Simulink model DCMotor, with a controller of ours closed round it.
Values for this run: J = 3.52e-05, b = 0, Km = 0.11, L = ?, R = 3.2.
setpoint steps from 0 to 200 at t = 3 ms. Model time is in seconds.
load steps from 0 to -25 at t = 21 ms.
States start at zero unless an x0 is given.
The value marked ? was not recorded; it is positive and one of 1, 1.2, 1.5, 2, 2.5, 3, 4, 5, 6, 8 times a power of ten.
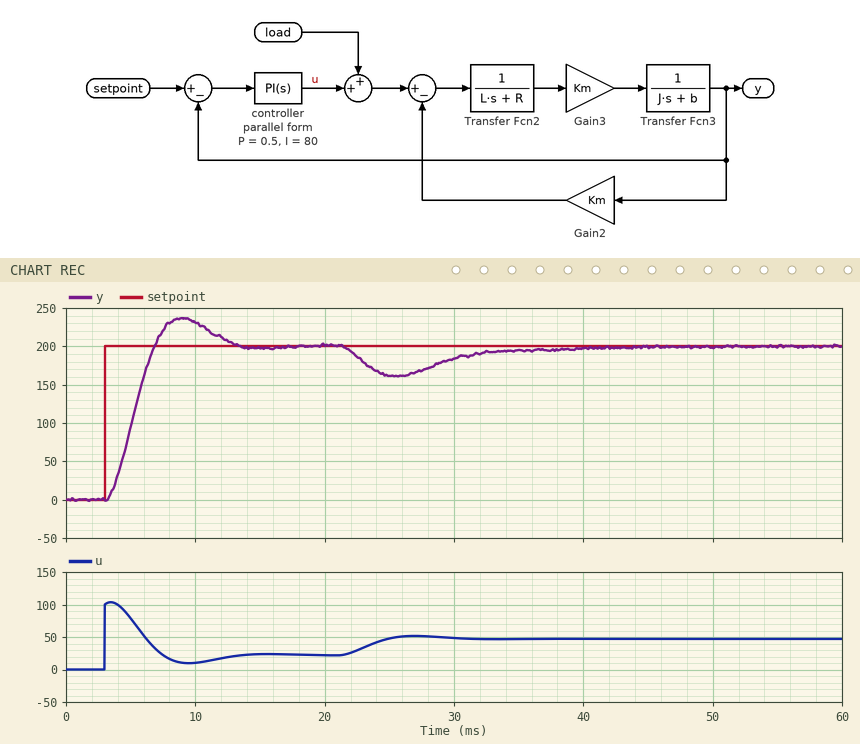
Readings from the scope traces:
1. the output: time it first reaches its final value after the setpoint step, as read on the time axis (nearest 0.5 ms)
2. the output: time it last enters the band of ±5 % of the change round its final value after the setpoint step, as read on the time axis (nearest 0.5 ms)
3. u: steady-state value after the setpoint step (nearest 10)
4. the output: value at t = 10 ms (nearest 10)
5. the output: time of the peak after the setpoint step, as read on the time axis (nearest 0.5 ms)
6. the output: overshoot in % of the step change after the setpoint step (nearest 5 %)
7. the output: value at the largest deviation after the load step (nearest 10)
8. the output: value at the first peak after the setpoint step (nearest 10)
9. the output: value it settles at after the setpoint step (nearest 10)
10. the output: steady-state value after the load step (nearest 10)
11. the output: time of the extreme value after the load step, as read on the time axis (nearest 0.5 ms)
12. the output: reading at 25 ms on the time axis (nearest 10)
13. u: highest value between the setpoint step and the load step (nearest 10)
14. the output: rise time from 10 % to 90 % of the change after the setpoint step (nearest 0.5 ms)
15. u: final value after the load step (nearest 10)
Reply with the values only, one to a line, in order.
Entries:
7.0 ms
12.0 ms
20
230
9.0 ms
20 %
160
240
200
200
25.5 ms
160
100
2.5 ms
50
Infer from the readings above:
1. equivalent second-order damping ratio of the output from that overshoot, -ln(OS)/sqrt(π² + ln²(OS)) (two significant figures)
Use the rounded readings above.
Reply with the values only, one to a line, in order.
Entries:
0.46
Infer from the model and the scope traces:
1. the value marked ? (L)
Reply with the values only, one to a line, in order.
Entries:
0.004
